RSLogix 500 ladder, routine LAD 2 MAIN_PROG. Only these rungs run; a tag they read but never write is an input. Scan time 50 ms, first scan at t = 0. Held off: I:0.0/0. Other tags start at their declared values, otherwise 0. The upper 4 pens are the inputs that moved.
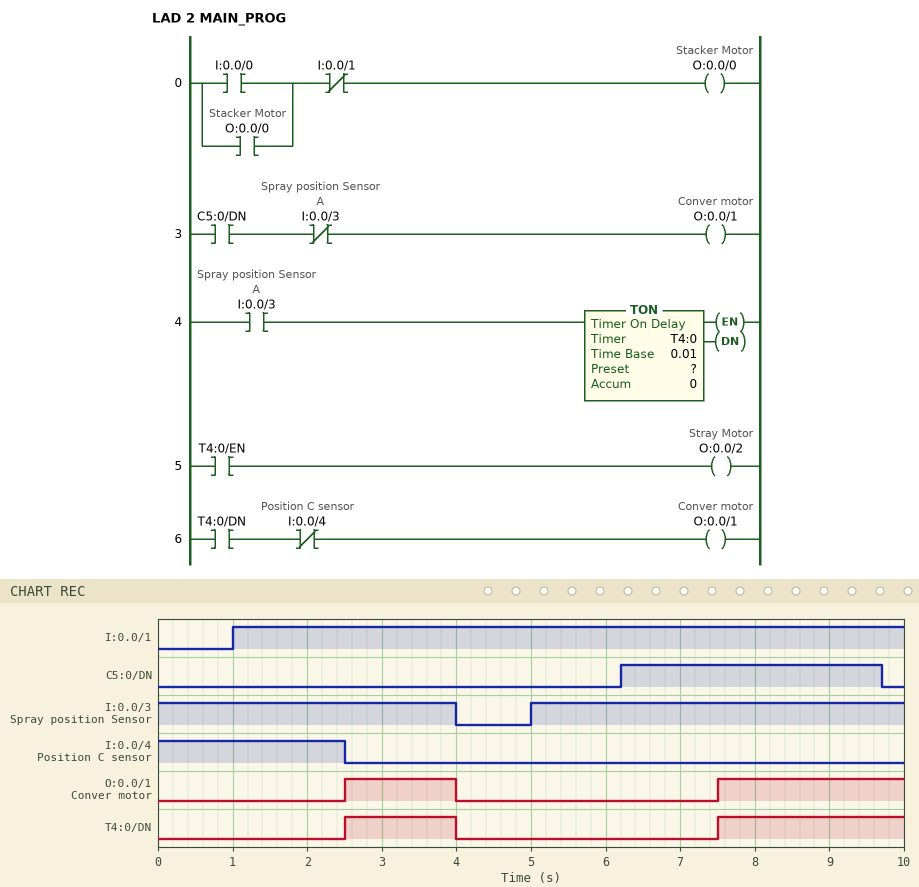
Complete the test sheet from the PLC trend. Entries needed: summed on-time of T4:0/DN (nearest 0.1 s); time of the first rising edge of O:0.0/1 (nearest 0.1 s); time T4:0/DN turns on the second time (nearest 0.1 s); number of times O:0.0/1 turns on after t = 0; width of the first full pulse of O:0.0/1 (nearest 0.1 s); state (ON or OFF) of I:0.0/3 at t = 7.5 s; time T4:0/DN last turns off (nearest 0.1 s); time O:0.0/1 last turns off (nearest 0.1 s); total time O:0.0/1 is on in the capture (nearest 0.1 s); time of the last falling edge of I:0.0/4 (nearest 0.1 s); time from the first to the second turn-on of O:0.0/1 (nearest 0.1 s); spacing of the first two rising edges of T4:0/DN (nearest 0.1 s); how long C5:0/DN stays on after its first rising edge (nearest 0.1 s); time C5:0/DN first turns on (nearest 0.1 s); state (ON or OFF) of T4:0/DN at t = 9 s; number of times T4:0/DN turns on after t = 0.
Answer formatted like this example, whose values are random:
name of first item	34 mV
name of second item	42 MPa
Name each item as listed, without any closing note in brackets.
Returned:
summed on-time of T4:0/DN	4.0 s
time of the first rising edge of O:0.0/1	2.5 s
time T4:0/DN turns on the second time	7.5 s
number of times O:0.0/1 turns on after t = 0	2
width of the first full pulse of O:0.0/1	1.5 s
state (ON or OFF) of I:0.0/3 at t = 7.5 s	ON
time T4:0/DN last turns off	4.0 s
time O:0.0/1 last turns off	4.0 s
total time O:0.0/1 is on in the capture	4.0 s
time of the last falling edge of I:0.0/4	2.5 s
time from the first to the second turn-on of O:0.0/1	5.0 s
spacing of the first two rising edges of T4:0/DN	5.0 s
how long C5:0/DN stays on after its first rising edge	3.5 s
time C5:0/DN first turns on	6.2 s
state (ON or OFF) of T4:0/DN at t = 9 s	ON
number of times T4:0/DN turns on after t = 0	2
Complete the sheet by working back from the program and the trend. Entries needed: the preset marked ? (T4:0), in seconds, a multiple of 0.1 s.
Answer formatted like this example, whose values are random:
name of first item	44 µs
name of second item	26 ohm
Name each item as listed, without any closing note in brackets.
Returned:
the preset marked ? (T4:0), in seconds, a multiple of 0.1 s	2.5 s
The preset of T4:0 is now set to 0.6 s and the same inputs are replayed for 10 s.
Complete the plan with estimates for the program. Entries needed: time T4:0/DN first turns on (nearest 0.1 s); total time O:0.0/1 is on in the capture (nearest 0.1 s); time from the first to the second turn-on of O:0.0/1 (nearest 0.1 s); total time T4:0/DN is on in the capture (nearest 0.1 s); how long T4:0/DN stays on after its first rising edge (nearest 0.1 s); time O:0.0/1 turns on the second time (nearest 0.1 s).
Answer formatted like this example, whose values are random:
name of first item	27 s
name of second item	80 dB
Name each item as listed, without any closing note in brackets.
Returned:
time T4:0/DN first turns on	0.6 s
total time O:0.0/1 is on in the capture	5.9 s
time from the first to the second turn-on of O:0.0/1	3.1 s
total time T4:0/DN is on in the capture	7.8 s
how long T4:0/DN stays on after its first rising edge	3.4 s
time O:0.0/1 turns on the second time	5.6 s
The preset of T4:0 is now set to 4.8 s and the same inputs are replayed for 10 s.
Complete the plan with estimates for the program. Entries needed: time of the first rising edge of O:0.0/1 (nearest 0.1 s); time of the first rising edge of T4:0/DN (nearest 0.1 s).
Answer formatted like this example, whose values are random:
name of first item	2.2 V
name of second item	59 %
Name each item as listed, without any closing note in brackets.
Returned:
time of the first rising edge of O:0.0/1	9.8 s
time of the first rising edge of T4:0/DN	9.8 s
